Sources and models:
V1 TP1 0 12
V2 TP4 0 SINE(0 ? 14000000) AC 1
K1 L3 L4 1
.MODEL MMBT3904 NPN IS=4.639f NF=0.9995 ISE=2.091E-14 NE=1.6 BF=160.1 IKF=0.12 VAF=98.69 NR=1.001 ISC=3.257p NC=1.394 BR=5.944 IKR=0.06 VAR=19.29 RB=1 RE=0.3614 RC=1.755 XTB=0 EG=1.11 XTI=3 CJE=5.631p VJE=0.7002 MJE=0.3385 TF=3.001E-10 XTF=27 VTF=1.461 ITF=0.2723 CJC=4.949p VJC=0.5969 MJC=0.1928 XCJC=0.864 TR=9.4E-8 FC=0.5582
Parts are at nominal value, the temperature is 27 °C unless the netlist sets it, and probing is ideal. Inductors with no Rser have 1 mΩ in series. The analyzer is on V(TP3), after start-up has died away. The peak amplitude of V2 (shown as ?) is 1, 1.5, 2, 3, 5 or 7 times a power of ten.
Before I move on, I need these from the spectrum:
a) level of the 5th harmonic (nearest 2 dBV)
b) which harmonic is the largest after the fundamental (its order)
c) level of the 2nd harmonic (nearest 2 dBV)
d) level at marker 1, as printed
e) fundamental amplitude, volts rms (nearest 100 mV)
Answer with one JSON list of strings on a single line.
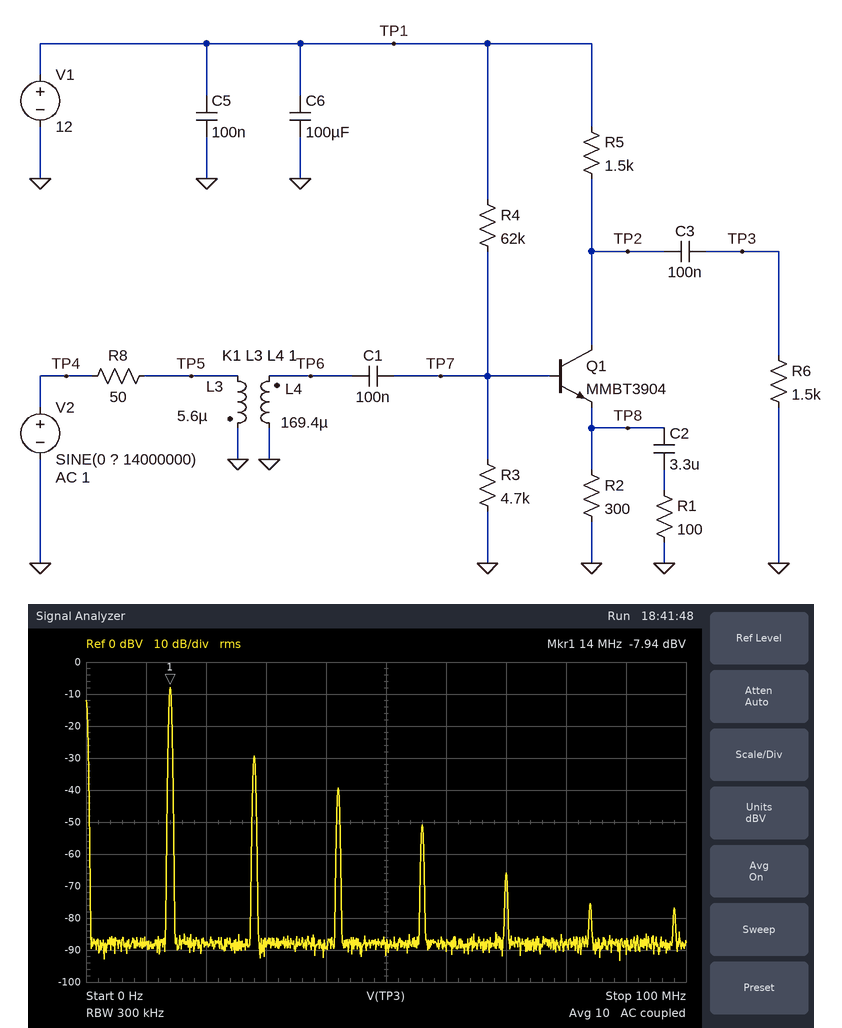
["-66 dBV", "2", "-30 dBV", "-7.94 dBV", "400 mV"]
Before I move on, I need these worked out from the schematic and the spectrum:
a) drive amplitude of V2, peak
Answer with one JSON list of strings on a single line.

["70 mV"]
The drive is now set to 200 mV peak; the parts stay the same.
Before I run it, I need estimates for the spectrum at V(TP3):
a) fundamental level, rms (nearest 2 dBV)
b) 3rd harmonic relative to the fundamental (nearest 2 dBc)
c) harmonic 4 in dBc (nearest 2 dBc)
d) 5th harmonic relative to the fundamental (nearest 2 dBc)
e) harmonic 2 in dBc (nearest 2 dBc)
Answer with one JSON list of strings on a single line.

["0 dBV", "-24 dBc", "-58 dBc", "-36 dBc", "-14 dBc"]
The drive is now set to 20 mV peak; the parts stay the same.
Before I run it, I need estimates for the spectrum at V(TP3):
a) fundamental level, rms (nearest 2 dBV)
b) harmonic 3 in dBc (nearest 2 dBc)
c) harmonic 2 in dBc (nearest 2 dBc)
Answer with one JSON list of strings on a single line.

["-18 dBV", "-54 dBc", "-34 dBc"]
